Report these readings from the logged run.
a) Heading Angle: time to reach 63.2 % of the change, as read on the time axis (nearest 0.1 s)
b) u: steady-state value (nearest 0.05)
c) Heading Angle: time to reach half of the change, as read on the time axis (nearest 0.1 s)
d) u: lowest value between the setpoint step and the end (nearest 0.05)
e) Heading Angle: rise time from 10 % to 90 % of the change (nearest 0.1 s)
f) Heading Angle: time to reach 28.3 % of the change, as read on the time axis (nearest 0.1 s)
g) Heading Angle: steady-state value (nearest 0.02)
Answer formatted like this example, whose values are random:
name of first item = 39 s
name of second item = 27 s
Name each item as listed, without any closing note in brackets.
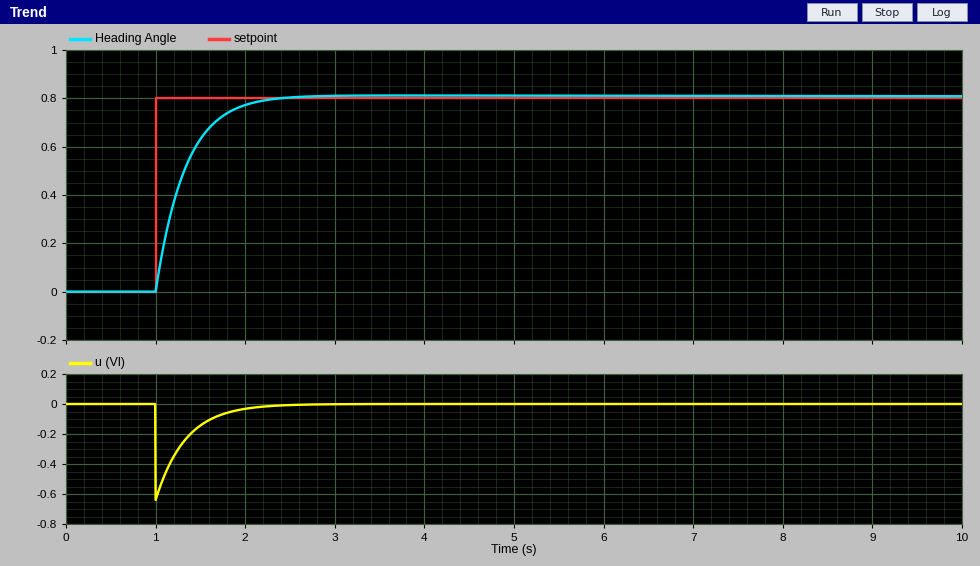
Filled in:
Heading Angle: time to reach 63.2 % of the change, as read on the time axis = 1.3 s
u: steady-state value = 0.00
Heading Angle: time to reach half of the change, as read on the time axis = 1.2 s
u: lowest value between the setpoint step and the end = -0.65
Heading Angle: rise time from 10 % to 90 % of the change = 0.7 s
Heading Angle: time to reach 28.3 % of the change, as read on the time axis = 1.1 s
Heading Angle: steady-state value = 0.80
